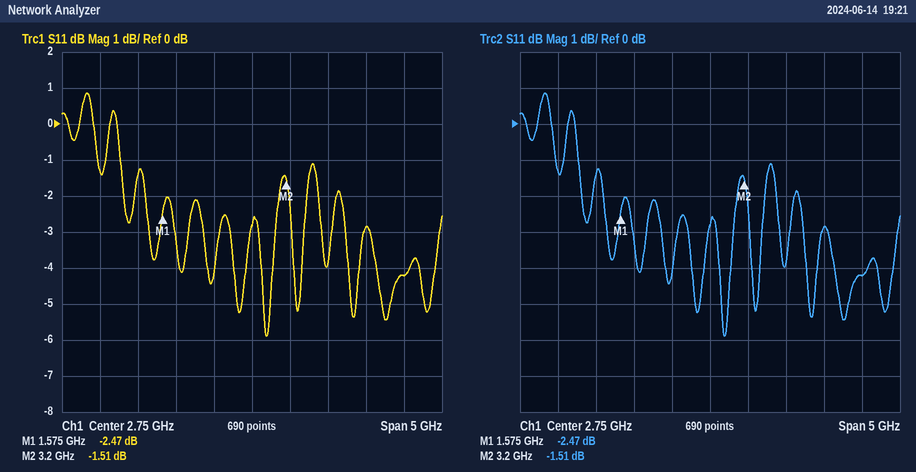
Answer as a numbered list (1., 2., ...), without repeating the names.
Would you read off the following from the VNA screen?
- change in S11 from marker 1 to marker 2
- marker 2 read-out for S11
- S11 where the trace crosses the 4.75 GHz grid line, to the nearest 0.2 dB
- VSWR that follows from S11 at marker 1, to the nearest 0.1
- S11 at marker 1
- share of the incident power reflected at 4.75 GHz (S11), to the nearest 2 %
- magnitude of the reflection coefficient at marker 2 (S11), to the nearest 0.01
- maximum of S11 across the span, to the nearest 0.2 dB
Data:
1. 0.96 dB
2. -1.51 dB
3. -4.2 dB
4. 7.1
5. -2.47 dB
6. 38 %
7. 0.84
8. 0.8 dB
